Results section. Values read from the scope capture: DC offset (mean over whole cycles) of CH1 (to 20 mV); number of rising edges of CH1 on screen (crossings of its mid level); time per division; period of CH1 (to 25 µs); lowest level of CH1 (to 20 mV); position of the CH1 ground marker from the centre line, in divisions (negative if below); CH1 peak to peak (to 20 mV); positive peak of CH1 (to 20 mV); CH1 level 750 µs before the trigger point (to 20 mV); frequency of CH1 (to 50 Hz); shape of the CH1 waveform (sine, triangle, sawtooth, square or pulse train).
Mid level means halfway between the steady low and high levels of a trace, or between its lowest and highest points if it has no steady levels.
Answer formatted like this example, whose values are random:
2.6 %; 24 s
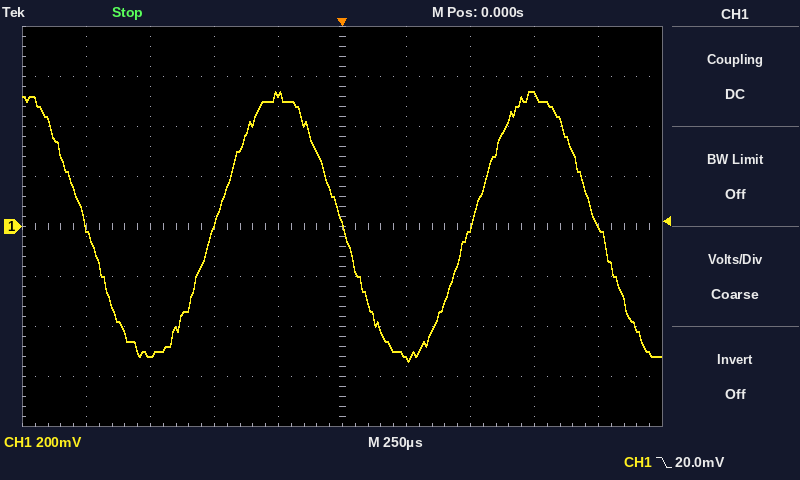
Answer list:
0 mV; 2; 250 µs; 1.000 ms; -540 mV; 0.0 div; 1.08 V; 540 mV; -520 mV; 1.00 kHz; sine
